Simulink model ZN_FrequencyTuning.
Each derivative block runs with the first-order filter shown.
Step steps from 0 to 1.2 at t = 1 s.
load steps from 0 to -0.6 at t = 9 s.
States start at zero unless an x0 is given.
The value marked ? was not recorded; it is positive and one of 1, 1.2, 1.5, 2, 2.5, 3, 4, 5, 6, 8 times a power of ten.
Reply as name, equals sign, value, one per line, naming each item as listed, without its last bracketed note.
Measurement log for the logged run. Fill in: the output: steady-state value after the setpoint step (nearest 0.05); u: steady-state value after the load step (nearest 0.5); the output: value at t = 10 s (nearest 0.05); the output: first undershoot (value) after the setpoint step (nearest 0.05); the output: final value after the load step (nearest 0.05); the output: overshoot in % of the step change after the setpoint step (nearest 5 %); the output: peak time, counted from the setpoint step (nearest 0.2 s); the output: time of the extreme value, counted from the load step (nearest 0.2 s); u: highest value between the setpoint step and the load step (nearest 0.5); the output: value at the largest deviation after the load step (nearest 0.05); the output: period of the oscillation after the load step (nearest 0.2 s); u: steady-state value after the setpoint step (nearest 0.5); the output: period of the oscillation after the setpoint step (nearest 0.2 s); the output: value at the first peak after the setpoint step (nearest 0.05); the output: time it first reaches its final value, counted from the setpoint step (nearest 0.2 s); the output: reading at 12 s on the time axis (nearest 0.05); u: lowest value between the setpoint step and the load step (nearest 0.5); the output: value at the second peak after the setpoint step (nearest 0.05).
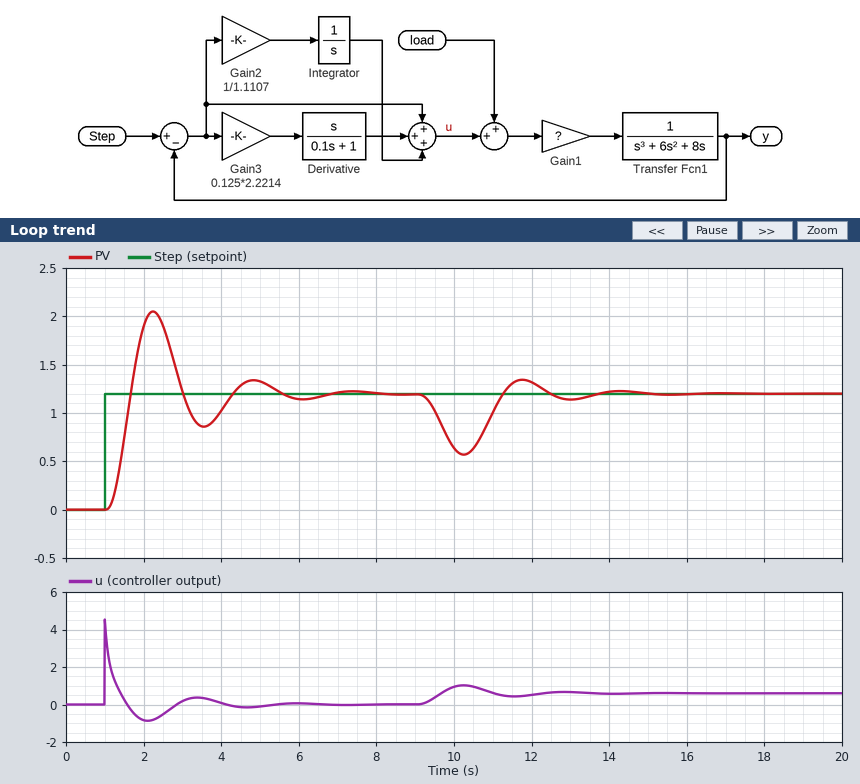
the output: steady-state value after the setpoint step = 1.20
u: steady-state value after the load step = 0.5
the output: value at t = 10 s = 0.65
the output: first undershoot (value) after the setpoint step = 0.85
the output: final value after the load step = 1.20
the output: overshoot in % of the step change after the setpoint step = 70 %
the output: peak time, counted from the setpoint step = 1.2 s
the output: time of the extreme value, counted from the load step = 1.2 s
u: highest value between the setpoint step and the load step = 4.5
the output: value at the largest deviation after the load step = 0.55
the output: period of the oscillation after the load step = 2.8 s
u: steady-state value after the setpoint step = 0.0
the output: period of the oscillation after the setpoint step = 2.6 s
the output: value at the first peak after the setpoint step = 2.05
the output: time it first reaches its final value, counted from the setpoint step = 0.6 s
the output: reading at 12 s on the time axis = 1.30
u: lowest value between the setpoint step and the load step = -1.0
the output: value at the second peak after the setpoint step = 1.35
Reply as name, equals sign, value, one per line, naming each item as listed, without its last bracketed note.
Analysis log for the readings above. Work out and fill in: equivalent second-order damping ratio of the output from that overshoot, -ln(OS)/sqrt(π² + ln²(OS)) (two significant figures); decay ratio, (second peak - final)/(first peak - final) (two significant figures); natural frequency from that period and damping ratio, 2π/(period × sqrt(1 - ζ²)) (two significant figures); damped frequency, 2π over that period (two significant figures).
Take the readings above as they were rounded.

equivalent second-order damping ratio of the output from that overshoot, -ln(OS)/sqrt(π² + ln²(OS)) = 0.11
decay ratio, (second peak - final)/(first peak - final) = 0.18
natural frequency from that period and damping ratio, 2π/(period × sqrt(1 - ζ²)) = 2.4 rad/s
damped frequency, 2π over that period = 2.4 rad/s
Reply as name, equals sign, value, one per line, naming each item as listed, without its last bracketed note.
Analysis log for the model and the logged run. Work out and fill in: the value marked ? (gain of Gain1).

the value marked ? = 30
